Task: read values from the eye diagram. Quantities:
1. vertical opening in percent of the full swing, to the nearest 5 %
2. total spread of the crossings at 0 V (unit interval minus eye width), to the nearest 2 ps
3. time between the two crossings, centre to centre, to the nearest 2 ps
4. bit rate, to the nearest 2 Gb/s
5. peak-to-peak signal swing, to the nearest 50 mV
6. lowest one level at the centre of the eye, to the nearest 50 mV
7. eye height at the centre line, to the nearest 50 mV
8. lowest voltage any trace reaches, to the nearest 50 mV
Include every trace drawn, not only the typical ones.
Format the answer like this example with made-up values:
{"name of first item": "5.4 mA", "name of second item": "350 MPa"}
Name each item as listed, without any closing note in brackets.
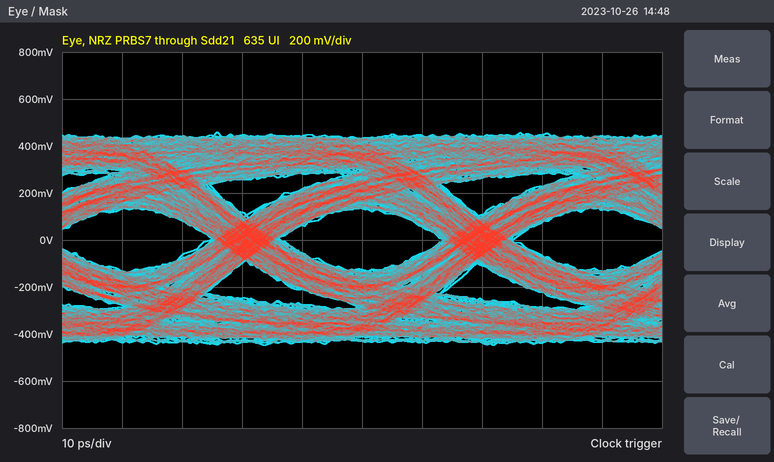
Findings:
{"vertical opening in percent of the full swing, to the nearest 5 %": "30 %", "total spread of the crossings at 0 V (unit interval minus eye width), to the nearest 2 ps": "12 ps", "time between the two crossings, centre to centre, to the nearest 2 ps": "38 ps", "bit rate, to the nearest 2 Gb/s": "26 Gb/s", "peak-to-peak signal swing, to the nearest 50 mV": "900 mV", "lowest one level at the centre of the eye, to the nearest 50 mV": "150 mV", "eye height at the centre line, to the nearest 50 mV": "250 mV", "lowest voltage any trace reaches, to the nearest 50 mV": "-450 mV"}
